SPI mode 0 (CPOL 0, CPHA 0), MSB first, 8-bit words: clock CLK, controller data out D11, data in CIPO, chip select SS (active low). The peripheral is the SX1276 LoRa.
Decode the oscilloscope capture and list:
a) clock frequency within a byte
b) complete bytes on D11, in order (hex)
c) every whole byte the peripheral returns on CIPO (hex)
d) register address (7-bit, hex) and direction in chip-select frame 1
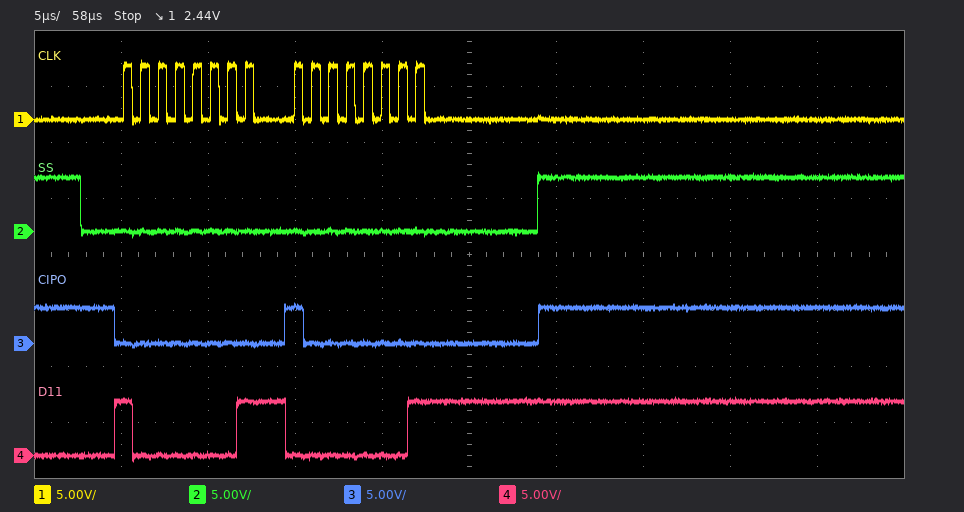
1 MHz
0x81 0x01
0x00 0x80
0x01 write
